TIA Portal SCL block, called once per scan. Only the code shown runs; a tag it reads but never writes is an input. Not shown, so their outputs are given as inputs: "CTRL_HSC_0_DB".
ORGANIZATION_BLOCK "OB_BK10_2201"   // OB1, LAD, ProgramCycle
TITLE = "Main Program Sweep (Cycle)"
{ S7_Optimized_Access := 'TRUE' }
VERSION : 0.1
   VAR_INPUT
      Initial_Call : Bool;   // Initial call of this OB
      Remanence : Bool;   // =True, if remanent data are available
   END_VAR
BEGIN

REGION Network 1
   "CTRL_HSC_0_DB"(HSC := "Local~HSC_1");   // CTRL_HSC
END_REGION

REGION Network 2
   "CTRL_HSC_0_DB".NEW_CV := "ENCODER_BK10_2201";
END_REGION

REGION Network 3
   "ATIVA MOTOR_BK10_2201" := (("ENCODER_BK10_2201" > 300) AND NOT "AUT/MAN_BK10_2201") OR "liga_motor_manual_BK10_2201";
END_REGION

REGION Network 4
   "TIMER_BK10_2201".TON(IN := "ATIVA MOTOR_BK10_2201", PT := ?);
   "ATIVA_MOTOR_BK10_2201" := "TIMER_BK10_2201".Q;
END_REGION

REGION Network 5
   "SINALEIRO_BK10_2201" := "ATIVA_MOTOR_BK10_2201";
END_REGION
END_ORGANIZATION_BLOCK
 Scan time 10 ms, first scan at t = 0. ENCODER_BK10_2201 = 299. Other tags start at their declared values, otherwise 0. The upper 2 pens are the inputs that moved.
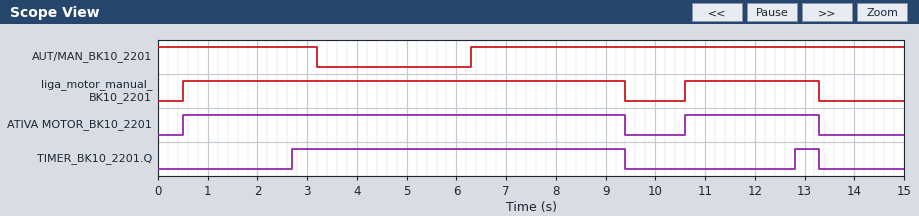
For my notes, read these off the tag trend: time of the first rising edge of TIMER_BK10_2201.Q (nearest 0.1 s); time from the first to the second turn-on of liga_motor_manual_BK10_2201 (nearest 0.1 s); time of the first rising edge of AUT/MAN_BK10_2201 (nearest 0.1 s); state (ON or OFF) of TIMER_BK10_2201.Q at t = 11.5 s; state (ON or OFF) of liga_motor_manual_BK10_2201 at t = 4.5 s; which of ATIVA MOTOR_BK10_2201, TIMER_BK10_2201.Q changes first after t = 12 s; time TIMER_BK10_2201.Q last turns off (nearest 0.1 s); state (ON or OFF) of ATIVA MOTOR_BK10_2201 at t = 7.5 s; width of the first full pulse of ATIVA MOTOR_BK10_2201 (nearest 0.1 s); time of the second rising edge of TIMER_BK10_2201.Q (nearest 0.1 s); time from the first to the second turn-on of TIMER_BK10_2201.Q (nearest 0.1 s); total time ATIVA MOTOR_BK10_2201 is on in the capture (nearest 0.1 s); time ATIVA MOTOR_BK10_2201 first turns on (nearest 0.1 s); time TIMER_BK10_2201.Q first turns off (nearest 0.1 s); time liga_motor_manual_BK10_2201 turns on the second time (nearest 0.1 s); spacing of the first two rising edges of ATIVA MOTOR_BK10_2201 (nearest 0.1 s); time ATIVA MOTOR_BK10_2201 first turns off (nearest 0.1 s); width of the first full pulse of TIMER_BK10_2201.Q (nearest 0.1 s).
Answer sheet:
2.7 s
10.1 s
6.3 s
OFF
ON
TIMER_BK10_2201.Q
13.3 s
ON
8.9 s
12.8 s
10.1 s
11.6 s
0.5 s
9.4 s
10.6 s
10.1 s
9.4 s
6.7 s
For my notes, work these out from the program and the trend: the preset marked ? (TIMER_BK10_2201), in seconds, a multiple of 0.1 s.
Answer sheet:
2.2 s
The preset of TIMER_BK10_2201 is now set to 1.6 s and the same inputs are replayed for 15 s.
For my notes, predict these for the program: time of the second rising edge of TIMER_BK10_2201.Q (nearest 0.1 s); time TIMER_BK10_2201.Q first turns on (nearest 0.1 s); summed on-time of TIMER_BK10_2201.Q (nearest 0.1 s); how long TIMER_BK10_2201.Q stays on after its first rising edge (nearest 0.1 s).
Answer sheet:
12.2 s
2.1 s
8.4 s
7.3 s
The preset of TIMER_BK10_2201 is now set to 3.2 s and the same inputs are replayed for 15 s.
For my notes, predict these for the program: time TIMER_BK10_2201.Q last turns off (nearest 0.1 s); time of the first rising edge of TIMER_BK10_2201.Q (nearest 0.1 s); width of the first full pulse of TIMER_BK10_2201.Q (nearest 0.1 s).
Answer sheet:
9.4 s
3.7 s
5.7 s
